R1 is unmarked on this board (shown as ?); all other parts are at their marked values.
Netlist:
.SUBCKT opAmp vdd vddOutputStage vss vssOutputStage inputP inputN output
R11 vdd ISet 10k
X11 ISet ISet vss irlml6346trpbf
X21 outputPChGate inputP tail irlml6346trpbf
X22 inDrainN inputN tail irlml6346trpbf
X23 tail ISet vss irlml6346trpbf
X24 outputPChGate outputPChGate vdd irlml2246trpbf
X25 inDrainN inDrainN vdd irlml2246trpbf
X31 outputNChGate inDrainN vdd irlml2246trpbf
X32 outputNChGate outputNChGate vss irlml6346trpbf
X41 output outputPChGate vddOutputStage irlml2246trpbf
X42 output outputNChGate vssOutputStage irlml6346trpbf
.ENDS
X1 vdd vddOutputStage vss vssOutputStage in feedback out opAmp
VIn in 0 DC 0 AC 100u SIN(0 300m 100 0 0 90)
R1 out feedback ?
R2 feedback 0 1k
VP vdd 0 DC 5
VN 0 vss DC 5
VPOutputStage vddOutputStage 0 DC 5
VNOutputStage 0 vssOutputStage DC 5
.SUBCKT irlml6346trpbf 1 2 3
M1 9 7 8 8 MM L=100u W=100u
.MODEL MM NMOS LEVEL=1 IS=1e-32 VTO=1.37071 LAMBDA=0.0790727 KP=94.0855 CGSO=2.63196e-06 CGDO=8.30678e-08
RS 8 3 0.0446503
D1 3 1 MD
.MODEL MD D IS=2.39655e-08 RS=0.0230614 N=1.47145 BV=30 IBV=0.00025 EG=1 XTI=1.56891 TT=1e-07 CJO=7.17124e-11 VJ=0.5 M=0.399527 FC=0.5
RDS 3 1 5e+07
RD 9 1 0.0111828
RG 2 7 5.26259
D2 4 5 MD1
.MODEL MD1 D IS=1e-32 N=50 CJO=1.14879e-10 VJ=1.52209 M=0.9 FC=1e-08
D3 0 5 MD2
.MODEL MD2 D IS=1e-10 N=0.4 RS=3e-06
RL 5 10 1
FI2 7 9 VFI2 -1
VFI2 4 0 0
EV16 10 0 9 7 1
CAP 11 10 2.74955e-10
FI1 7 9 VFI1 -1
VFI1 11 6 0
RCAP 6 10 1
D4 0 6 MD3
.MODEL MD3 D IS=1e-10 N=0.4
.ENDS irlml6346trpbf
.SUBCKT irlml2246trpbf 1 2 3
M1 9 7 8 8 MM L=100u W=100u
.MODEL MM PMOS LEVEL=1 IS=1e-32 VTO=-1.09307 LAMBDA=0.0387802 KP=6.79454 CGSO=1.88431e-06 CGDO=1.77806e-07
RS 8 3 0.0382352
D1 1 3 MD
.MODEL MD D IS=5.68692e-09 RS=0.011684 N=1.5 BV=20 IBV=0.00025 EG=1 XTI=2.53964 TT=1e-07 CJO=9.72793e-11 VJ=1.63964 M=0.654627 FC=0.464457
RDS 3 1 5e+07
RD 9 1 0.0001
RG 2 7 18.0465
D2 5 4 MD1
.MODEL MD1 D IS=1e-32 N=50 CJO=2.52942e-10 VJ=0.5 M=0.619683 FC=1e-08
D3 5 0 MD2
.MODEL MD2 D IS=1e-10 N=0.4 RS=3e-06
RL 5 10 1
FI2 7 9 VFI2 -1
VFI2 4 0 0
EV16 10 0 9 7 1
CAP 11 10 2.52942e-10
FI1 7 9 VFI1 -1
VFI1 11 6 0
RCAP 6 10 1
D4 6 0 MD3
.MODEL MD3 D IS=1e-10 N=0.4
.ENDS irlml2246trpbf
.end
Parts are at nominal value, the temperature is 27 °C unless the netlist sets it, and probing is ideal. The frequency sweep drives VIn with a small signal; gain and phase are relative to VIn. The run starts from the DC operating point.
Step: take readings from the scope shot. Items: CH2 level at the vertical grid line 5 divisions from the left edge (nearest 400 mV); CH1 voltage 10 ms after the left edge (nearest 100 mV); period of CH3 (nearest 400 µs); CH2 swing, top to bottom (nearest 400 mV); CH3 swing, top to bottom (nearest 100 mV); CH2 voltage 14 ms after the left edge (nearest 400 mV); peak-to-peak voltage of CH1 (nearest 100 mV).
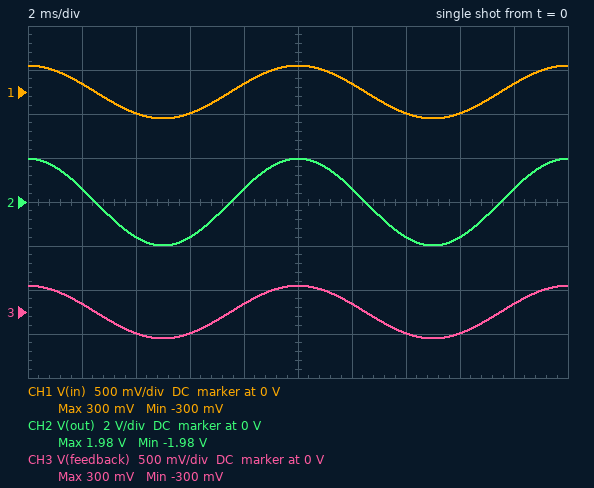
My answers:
2.0 V
300 mV
10.0 ms
4.0 V
600 mV
-1.6 V
600 mV
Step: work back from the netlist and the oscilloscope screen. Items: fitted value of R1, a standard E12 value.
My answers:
5.6 kΩ
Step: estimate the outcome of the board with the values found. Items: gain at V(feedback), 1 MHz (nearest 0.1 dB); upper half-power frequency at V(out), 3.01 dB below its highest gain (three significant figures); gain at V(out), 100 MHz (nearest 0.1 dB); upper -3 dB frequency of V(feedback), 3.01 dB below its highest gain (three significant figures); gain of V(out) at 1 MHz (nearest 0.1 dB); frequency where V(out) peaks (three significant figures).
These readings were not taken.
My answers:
0.1 dB
3.64 MHz
-17.2 dB
3.57 MHz
17.3 dB
3.50 MHz
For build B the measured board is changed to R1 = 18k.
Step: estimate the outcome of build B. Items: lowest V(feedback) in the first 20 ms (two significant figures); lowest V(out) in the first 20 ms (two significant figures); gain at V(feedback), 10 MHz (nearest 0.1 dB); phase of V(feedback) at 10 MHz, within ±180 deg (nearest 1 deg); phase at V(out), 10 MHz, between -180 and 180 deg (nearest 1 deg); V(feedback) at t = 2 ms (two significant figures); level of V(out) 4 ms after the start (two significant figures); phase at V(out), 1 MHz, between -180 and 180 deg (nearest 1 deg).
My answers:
-260 mV
-5.0 V
-1.7 dB
-2 deg
-116 deg
92 mV
-4.6 V
4 deg
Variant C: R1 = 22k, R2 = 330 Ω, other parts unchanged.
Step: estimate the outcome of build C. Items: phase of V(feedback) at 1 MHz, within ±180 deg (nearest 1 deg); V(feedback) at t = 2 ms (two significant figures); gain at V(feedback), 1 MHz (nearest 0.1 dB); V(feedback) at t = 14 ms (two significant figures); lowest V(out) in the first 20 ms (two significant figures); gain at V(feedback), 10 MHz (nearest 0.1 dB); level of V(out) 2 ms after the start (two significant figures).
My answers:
-38 deg
74 mV
-1.3 dB
-74 mV
-5.0 V
-2.0 dB
5.0 V
